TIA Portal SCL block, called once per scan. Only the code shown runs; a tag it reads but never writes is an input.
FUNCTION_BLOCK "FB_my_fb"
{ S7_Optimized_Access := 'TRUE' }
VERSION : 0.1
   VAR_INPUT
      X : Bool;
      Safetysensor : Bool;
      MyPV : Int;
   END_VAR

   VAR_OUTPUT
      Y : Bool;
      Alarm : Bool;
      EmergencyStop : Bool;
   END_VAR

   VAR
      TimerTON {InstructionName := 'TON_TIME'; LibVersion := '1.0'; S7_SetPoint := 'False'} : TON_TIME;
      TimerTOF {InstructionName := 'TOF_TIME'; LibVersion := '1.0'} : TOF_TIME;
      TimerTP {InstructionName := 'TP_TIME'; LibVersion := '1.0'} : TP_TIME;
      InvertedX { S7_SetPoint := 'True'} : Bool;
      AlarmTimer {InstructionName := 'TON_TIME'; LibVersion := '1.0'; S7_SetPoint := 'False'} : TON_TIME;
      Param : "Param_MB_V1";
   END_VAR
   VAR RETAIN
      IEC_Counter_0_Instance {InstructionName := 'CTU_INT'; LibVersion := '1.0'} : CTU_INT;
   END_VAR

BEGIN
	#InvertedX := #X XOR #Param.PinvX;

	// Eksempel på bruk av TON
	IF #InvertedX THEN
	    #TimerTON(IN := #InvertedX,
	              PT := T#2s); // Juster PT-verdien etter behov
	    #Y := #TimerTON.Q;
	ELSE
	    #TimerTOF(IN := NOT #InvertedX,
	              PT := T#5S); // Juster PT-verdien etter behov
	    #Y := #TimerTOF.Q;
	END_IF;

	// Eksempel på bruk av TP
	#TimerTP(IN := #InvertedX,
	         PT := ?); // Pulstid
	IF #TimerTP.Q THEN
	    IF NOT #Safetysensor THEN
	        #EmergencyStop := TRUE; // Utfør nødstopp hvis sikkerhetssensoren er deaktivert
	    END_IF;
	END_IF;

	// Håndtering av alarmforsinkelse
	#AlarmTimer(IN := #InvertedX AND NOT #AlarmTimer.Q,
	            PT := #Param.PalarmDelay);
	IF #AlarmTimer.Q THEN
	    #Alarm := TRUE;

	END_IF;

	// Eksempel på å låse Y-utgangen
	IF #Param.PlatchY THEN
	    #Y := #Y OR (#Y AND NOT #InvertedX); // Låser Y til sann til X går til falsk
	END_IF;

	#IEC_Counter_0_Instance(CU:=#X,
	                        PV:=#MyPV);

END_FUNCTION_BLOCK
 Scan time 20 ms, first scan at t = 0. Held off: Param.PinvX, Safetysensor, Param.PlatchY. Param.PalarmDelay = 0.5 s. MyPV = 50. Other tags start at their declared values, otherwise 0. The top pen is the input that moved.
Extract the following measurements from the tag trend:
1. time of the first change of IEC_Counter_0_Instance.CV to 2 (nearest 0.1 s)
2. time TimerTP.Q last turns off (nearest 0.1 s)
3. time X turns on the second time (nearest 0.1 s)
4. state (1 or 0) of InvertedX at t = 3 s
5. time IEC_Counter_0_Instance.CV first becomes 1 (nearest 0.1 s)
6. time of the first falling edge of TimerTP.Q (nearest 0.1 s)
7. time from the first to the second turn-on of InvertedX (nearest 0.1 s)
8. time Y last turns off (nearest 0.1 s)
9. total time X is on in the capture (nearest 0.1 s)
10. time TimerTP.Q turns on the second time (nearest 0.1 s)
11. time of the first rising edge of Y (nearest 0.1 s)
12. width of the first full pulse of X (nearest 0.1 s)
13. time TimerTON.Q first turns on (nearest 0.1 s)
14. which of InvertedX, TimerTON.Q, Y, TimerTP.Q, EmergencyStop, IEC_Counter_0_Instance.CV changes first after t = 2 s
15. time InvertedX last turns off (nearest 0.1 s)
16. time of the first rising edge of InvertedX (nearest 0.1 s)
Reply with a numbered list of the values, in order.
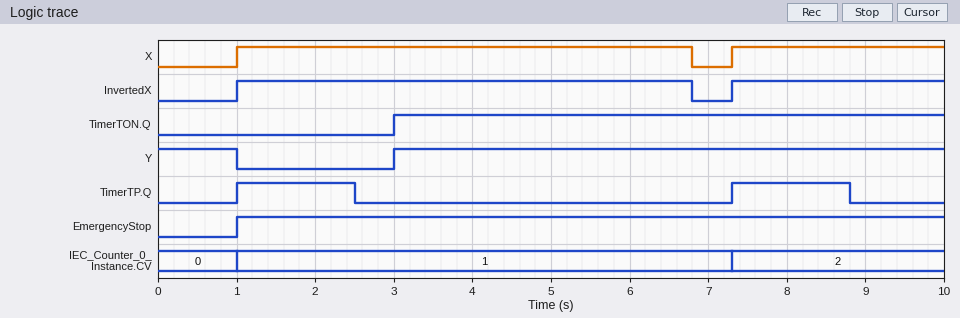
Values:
1. 7.3 s
2. 8.8 s
3. 7.3 s
4. 1
5. 1.0 s
6. 2.5 s
7. 6.3 s
8. 1.0 s
9. 8.5 s
10. 7.3 s
11. 3.0 s
12. 5.8 s
13. 3.0 s
14. TimerTP.Q
15. 6.8 s
16. 1.0 s
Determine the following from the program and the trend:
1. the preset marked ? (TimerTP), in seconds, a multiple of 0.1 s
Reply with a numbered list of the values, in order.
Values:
1. 1.5 s
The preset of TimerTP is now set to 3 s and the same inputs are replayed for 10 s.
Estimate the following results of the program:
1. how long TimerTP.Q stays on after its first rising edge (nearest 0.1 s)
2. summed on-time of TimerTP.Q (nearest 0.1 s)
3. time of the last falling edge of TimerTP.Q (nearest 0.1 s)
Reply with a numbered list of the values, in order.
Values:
1. 3.0 s
2. 5.7 s
3. 4.0 s
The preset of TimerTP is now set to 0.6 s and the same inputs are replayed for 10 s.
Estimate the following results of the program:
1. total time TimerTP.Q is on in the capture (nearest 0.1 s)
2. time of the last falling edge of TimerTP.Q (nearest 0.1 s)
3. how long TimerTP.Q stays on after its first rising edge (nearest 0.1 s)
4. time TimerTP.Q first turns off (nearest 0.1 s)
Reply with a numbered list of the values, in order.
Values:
1. 1.2 s
2. 7.9 s
3. 0.6 s
4. 1.6 s
